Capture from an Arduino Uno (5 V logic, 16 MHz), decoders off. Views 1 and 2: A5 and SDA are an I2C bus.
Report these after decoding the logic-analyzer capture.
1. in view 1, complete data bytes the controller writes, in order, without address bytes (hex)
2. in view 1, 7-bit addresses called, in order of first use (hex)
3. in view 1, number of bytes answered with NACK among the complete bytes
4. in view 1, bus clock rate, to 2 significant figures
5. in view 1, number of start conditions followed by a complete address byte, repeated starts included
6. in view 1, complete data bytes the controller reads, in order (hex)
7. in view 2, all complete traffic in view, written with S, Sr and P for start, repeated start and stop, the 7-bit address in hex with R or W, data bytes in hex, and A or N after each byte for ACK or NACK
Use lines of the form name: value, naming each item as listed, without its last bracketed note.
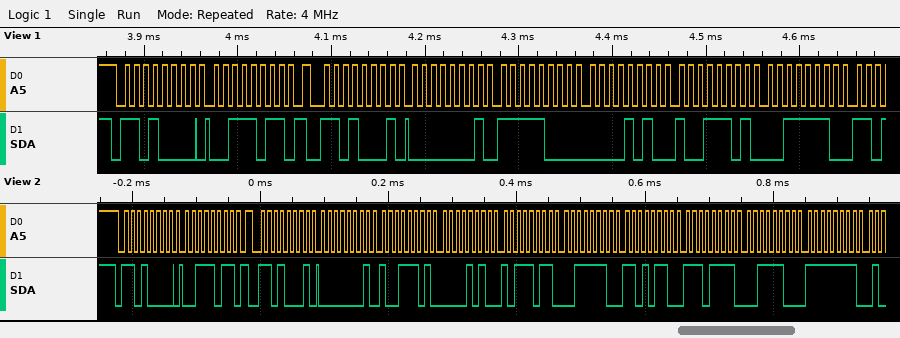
in view 1, complete data bytes the controller writes, in order, without address bytes: 3B
in view 1, 7-bit addresses called, in order of first use: 0x68
in view 1, number of bytes answered with NACK among the complete bytes: 0
in view 1, bus clock rate, to 2 significant figures: 100 kHz
in view 1, number of start conditions followed by a complete address byte, repeated starts included: 2
in view 1, complete data bytes the controller reads, in order: 01 F8 0A 9D 3E
in view 2, all complete traffic in view, written with S, Sr and P for start, repeated start and stop, the 7-bit address in hex with R or W, data bytes in hex, and A or N after each byte for ACK or NACK: S 68W A 3B A Sr 68R A 01 A 9D A 0A A BB A 3E A D6 A EF A 3C A FF A
